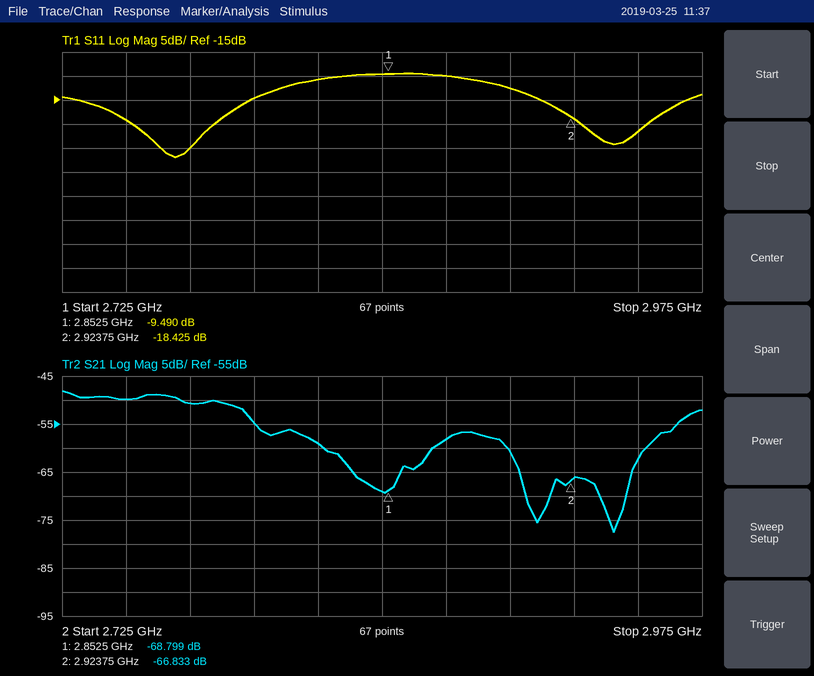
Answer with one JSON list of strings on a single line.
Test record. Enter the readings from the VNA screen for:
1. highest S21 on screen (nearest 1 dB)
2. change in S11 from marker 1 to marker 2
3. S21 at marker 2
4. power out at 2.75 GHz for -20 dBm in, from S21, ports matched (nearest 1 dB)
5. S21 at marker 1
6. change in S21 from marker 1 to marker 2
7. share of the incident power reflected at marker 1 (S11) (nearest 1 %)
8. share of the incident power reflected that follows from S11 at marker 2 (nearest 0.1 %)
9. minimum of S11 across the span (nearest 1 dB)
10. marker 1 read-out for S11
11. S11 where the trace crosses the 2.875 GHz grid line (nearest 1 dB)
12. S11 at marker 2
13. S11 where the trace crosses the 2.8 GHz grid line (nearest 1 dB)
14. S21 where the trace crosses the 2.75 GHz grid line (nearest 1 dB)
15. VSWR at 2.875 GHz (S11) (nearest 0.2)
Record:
["-48 dB", "-8.935 dB", "-66.833 dB", "-70 dBm", "-68.799 dB", "1.966 dB", "11 %", "1.4 %", "-27 dB", "-9.490 dB", "-10 dB", "-18.425 dB", "-15 dB", "-50 dB", "2.0"]
